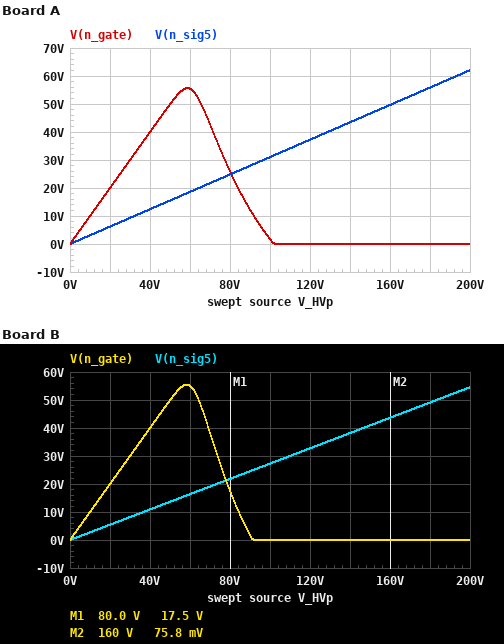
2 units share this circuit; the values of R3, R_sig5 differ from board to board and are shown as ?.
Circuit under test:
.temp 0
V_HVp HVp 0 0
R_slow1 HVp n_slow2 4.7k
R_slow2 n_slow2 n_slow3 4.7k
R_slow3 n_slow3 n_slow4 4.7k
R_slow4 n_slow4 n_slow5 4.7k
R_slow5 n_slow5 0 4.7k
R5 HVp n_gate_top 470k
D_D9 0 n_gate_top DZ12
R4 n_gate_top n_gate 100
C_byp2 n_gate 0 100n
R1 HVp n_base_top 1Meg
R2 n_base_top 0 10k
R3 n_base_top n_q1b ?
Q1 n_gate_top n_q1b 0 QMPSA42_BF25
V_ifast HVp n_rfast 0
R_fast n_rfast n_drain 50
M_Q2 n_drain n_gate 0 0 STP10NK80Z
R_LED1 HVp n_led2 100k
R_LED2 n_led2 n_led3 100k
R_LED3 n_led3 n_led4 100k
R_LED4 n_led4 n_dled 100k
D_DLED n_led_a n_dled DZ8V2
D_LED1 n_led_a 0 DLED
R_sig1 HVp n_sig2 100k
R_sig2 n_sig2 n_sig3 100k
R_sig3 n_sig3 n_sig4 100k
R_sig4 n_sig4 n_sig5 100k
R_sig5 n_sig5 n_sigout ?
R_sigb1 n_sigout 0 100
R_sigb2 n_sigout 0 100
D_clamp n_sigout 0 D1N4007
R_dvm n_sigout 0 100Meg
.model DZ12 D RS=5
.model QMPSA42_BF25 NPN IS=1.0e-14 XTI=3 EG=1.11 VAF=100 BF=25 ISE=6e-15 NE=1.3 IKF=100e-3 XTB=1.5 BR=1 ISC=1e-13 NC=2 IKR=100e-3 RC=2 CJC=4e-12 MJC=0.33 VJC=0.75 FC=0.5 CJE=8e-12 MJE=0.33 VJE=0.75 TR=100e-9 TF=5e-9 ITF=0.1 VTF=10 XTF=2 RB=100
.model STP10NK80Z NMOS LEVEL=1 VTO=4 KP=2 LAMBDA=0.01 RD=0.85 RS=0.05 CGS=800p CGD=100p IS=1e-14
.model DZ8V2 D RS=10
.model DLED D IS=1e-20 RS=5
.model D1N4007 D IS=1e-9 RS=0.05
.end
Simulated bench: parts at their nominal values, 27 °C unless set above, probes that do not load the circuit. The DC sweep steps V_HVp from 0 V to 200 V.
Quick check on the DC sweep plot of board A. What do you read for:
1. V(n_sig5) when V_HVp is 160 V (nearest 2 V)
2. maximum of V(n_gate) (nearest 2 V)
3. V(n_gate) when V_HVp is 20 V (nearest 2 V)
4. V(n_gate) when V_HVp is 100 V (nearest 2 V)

50 V
56 V
20 V
2 V
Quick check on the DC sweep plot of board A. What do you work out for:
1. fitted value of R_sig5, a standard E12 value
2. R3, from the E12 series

180 kΩ
22 kΩ
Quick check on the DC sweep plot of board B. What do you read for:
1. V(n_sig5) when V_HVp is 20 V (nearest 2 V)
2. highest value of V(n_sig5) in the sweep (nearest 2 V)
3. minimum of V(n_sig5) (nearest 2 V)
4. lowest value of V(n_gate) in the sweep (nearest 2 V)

6 V
54 V
0 V
0 V
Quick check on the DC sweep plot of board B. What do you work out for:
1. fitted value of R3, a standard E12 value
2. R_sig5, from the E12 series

15 kΩ
150 kΩ
